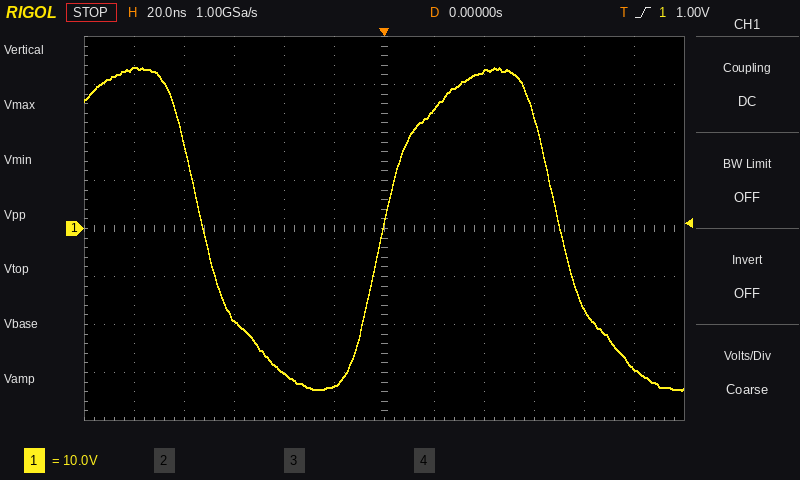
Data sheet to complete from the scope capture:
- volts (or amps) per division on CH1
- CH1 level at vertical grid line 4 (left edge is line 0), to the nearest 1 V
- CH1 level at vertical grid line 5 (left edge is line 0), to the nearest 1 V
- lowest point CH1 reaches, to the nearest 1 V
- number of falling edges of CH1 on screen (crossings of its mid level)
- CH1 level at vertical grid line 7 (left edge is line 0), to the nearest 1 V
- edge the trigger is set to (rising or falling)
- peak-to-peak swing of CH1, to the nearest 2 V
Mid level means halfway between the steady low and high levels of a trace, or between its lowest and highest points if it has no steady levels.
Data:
10 V
-30 V
-33 V
-34 V
2
25 V
rising
68 V
